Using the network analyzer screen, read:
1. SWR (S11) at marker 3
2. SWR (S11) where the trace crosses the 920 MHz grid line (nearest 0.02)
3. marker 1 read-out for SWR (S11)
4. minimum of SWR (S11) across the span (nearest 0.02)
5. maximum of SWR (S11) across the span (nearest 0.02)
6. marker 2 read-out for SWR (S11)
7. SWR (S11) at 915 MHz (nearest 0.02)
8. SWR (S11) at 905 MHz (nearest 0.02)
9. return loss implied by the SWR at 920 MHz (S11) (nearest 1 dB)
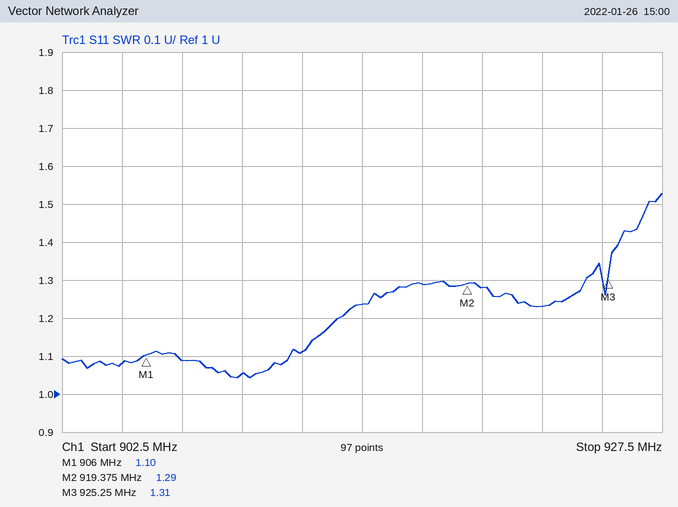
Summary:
1.31
1.28
1.10
1.04
1.52
1.29
1.24
1.08
18 dB
